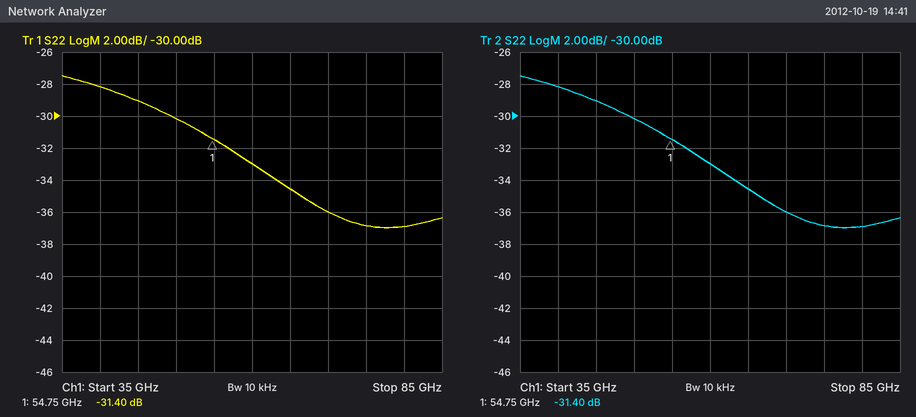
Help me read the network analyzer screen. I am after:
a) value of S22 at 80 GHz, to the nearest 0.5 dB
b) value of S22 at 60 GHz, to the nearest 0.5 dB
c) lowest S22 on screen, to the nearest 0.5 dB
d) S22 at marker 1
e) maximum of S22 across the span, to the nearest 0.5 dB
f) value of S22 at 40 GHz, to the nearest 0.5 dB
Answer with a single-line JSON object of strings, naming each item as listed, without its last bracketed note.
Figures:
{"value of S22 at 80 GHz, to the nearest 0.5 dB": "-37.0 dB", "value of S22 at 60 GHz, to the nearest 0.5 dB": "-33.0 dB", "lowest S22 on screen, to the nearest 0.5 dB": "-37.0 dB", "S22 at marker 1": "-31.40 dB", "maximum of S22 across the span, to the nearest 0.5 dB": "-27.5 dB", "value of S22 at 40 GHz, to the nearest 0.5 dB": "-28.0 dB"}
